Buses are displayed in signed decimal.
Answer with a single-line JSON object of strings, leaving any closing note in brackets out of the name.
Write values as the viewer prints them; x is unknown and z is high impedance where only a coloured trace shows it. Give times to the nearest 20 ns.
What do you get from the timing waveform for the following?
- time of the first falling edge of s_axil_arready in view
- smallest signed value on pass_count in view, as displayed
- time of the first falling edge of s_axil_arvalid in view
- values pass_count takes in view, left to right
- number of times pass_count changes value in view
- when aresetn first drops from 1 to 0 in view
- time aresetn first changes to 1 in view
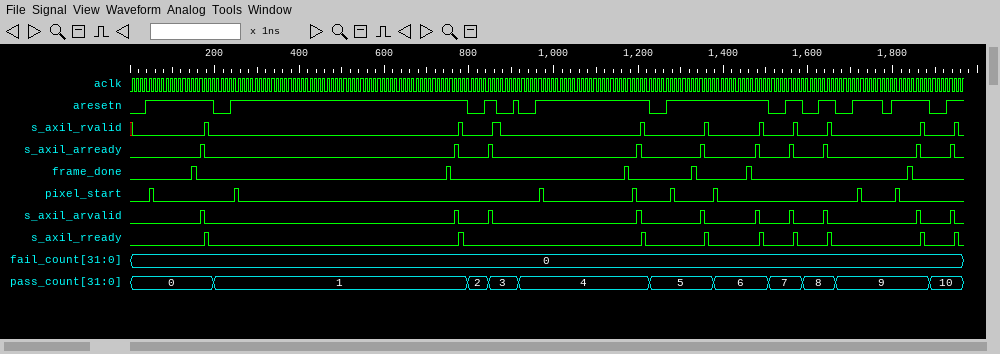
{"time of the first falling edge of s_axil_arready in view": "180 ns", "smallest signed value on pass_count in view, as displayed": "0", "time of the first falling edge of s_axil_arvalid in view": "180 ns", "values pass_count takes in view, left to right": "0, 1, 2, 3, 4, 5, 6, 7, 8, 9, 10", "number of times pass_count changes value in view": "10", "when aresetn first drops from 1 to 0 in view": "200 ns", "time aresetn first changes to 1 in view": "40 ns"}
